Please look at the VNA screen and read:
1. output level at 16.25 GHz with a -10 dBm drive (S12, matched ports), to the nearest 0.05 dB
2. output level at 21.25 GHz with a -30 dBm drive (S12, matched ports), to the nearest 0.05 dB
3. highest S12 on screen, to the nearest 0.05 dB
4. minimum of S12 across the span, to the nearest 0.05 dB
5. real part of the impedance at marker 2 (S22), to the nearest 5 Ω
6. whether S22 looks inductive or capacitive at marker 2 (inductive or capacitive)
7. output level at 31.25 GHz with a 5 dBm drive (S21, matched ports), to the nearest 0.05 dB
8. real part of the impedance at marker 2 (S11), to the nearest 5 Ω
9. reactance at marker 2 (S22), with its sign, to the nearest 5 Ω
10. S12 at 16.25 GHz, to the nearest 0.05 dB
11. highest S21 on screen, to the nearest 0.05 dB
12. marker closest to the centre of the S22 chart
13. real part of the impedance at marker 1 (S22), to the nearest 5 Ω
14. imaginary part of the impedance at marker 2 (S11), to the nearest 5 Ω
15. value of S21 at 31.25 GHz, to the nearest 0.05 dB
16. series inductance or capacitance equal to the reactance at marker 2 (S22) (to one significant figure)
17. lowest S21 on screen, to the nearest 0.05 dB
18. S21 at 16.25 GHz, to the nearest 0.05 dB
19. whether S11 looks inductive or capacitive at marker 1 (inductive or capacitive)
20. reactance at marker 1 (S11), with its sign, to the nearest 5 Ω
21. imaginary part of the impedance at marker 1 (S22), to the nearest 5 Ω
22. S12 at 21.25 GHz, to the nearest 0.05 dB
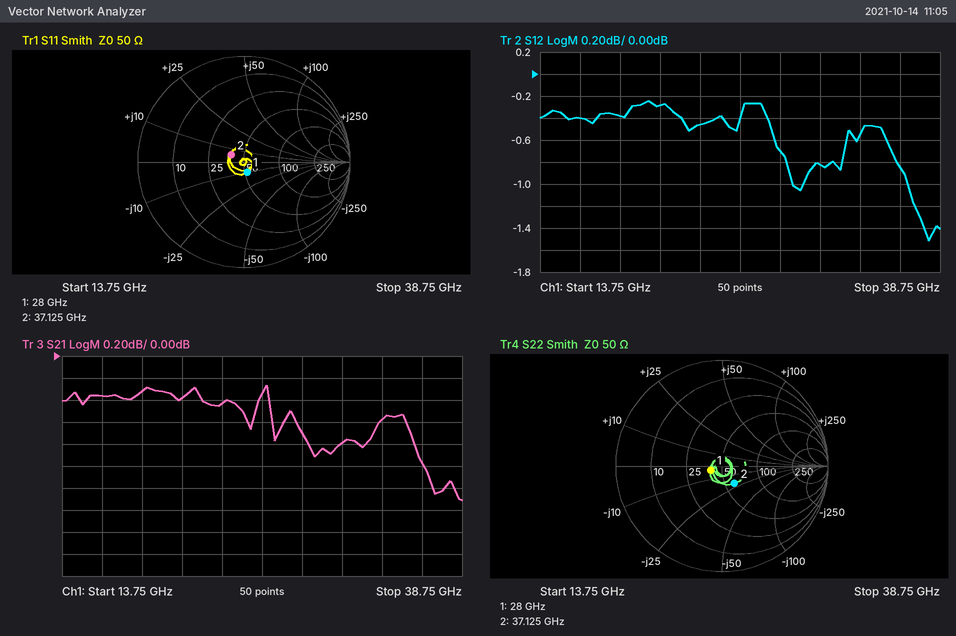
-10.40 dBm
-30.30 dBm
-0.25 dB
-1.50 dB
60 Ω
capacitive
4.20 dBm
40 Ω
-20 Ω
-0.40 dB
-0.25 dB
marker 1
40 Ω
+5 Ω
-0.80 dB
200 fF
-1.30 dB
-0.35 dB
capacitive
-10 Ω
-5 Ω
-0.30 dB
